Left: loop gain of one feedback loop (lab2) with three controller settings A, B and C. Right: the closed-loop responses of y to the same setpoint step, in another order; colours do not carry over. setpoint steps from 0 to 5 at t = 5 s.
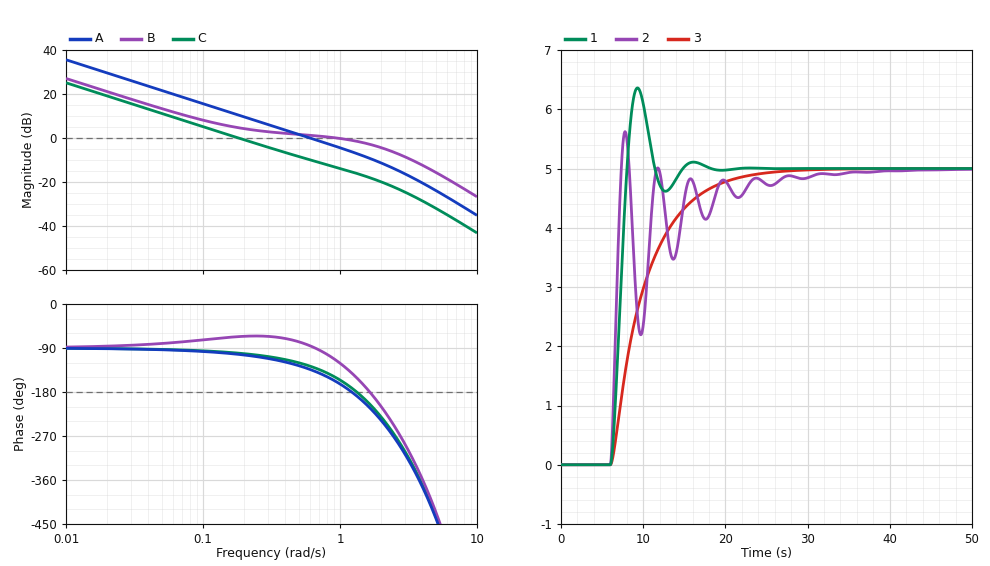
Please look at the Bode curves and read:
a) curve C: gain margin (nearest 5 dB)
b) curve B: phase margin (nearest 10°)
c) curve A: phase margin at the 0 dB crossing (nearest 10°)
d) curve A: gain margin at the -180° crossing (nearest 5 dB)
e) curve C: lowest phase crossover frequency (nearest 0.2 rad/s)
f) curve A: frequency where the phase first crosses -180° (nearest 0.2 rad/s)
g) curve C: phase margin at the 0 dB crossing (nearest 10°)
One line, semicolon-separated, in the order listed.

15 dB; 60°; 50°; 5 dB; 1.4 rad/s; 1.2 rad/s; 80°
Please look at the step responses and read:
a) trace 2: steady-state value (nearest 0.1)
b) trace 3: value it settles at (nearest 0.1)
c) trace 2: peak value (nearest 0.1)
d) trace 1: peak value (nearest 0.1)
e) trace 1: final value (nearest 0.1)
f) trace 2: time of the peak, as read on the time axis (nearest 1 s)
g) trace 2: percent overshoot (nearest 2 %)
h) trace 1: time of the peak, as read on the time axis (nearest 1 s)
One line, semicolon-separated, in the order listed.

5.0; 5.0; 5.6; 6.4; 5.0; 8 s; 12 %; 9 s
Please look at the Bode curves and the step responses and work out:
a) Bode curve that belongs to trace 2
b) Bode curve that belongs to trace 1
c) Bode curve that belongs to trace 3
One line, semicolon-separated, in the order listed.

B; A; C
